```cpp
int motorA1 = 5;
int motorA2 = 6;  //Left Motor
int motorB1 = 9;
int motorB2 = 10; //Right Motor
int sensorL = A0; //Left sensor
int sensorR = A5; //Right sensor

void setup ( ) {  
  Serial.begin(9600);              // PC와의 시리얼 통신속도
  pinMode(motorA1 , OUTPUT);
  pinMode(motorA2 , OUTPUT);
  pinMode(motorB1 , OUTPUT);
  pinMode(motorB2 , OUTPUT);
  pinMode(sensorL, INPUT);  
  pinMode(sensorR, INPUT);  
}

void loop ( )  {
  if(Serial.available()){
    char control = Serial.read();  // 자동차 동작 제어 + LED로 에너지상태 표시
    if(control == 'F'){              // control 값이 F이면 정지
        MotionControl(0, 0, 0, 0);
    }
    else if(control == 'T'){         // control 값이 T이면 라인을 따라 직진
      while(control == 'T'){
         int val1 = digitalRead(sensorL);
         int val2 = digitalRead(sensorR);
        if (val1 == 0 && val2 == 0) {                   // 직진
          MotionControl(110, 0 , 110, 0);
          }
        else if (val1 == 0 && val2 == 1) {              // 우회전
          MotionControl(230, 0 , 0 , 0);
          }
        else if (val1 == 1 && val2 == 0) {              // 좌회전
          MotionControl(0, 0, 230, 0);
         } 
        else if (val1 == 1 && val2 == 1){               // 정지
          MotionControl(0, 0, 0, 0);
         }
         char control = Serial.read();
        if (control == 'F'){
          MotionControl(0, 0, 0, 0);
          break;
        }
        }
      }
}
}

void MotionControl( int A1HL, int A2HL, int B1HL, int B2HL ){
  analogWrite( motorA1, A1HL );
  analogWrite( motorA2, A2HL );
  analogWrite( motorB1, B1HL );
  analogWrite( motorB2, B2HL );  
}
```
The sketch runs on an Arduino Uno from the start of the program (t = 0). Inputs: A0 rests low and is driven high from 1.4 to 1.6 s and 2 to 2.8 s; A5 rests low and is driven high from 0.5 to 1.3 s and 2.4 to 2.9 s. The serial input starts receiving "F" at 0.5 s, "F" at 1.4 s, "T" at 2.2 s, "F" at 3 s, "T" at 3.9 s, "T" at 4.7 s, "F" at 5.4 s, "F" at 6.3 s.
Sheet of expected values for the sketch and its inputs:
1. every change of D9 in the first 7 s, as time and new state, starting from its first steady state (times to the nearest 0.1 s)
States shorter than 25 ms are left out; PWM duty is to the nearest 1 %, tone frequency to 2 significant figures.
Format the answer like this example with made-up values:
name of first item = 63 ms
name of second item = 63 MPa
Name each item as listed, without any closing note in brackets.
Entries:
every change of D9 in the first 7 s, as time and new state, starting from its first steady state = 0 s low; 2.2 s PWM 90 %; 2.4 s low; 2.9 s PWM 43 %; 3 s low; 3.9 s PWM 43 %; 5.4 s low
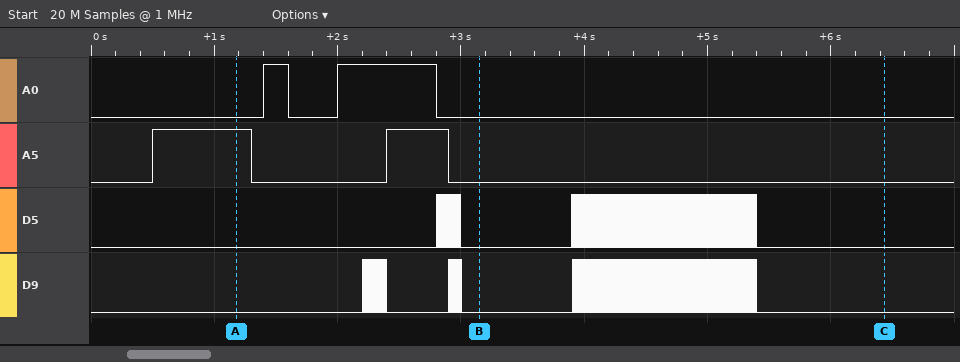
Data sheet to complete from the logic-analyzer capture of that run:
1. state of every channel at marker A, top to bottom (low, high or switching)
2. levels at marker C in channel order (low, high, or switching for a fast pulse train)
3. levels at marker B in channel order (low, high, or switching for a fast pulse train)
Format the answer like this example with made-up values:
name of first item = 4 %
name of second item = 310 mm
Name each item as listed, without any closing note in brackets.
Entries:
state of every channel at marker A, top to bottom = A0 low, A5 high, D5 low, D9 low
levels at marker C in channel order = A0 low, A5 low, D5 low, D9 low
levels at marker B in channel order = A0 low, A5 low, D5 low, D9 low
